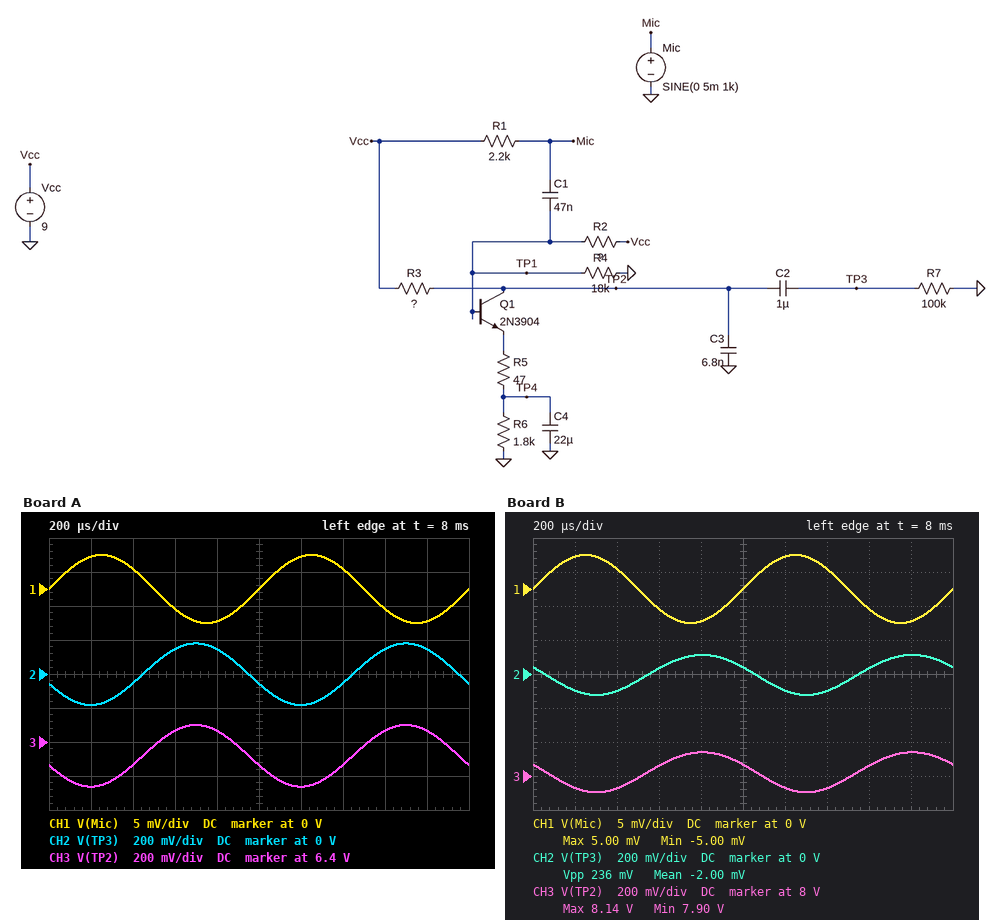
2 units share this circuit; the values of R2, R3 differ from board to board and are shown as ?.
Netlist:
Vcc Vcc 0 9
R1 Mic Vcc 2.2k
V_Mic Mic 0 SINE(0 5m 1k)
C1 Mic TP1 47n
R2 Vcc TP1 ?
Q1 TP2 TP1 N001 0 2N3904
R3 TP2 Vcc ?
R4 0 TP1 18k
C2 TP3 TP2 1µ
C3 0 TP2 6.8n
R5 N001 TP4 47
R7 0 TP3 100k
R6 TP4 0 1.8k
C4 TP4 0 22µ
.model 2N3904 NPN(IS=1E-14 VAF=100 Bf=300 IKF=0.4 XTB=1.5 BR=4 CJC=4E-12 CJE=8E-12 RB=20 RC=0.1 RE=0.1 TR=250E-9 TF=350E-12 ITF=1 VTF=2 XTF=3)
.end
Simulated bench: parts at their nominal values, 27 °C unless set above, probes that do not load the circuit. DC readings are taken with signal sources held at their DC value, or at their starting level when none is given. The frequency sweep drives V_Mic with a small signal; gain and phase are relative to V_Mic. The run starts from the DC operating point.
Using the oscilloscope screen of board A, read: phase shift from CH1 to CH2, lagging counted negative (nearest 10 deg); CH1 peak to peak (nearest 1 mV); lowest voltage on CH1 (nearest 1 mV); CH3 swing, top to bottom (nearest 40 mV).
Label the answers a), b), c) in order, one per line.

a) -160 deg
b) 10 mV
c) -5 mV
d) 360 mV
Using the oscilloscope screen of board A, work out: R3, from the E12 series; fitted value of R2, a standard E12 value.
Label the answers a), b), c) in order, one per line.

a) 3.3 kΩ
b) 56 kΩ
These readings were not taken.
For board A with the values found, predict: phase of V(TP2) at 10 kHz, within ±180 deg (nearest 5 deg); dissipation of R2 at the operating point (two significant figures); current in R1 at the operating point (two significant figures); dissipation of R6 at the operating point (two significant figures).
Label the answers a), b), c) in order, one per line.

a) 130 deg
b) 840 µW
c) 4.1 mA
d) 1.2 mW
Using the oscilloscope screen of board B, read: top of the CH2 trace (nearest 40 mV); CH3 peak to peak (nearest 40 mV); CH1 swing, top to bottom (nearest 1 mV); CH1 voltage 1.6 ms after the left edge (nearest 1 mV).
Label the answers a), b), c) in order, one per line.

a) 120 mV
b) 240 mV
c) 10 mV
d) -3 mV
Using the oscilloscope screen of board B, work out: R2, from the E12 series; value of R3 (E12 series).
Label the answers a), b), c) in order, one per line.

a) 220 kΩ
b) 18 kΩ
